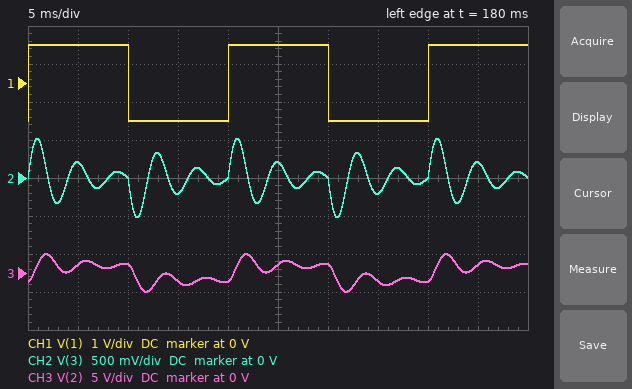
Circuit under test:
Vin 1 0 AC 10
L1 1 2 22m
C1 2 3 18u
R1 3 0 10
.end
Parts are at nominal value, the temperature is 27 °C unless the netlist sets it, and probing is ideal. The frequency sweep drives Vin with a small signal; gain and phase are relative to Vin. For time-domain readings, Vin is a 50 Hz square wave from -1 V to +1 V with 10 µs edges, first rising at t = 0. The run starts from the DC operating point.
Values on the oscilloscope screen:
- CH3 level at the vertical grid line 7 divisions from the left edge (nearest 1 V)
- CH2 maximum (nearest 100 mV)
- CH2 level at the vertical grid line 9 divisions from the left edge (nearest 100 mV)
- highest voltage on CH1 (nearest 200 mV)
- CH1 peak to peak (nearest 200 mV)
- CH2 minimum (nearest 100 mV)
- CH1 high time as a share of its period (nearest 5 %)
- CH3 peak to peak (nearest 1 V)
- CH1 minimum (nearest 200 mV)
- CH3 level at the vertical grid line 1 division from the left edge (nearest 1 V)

-1 V
500 mV
200 mV
1.0 V
2.0 V
-500 mV
50 %
5 V
-1.0 V
1 V
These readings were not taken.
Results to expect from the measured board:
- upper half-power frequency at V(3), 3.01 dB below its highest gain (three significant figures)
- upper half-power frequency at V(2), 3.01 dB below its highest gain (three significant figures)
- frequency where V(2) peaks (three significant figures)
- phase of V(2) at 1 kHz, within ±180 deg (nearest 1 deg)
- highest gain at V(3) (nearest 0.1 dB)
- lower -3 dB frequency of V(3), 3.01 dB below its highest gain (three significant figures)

292 Hz
283 Hz
248 Hz
-127 deg
0 dB
219 Hz
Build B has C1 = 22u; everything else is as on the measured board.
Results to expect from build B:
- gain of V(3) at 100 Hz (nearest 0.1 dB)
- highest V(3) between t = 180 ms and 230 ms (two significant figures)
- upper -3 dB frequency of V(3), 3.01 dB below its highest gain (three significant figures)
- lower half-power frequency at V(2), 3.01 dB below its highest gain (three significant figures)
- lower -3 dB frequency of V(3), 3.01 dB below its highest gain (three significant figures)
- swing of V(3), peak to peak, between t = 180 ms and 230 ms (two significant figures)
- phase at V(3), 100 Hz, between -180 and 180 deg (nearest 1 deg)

-15.5 dB
500 mV
268 Hz
184 Hz
195 Hz
990 mV
80 deg
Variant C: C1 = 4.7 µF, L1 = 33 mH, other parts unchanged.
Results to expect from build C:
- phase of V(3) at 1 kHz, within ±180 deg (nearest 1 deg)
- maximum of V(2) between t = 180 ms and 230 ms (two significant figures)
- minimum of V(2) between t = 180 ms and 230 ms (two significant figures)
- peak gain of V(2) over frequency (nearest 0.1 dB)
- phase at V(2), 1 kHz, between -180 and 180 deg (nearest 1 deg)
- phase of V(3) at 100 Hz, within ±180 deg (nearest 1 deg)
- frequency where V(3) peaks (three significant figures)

-87 deg
2.4 V
-2.4 V
18.5 dB
-160 deg
88 deg
404 Hz
